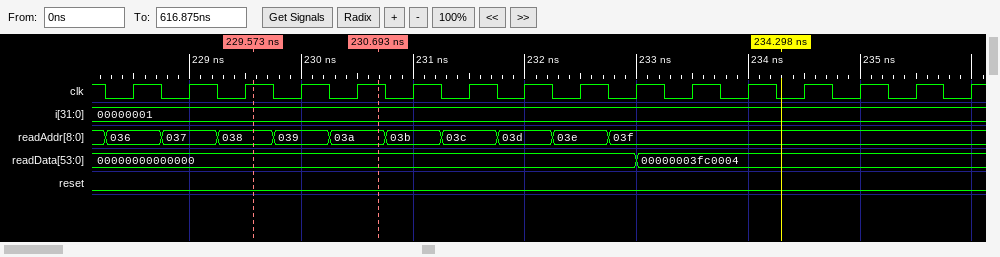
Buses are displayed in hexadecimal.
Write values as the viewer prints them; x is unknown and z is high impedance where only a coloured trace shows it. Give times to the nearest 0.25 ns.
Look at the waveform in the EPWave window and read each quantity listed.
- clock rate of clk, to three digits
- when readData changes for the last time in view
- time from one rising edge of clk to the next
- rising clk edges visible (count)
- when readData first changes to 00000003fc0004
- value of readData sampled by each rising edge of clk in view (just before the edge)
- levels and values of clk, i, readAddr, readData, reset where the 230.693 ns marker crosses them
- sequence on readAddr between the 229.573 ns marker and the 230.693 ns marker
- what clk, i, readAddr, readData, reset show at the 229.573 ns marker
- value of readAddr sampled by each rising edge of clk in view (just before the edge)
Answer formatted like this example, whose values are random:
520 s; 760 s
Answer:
2.00 GHz; 233 ns; 0.5 ns; 16; 233 ns; 00000000000000, 00000000000000, 00000000000000, 00000000000000, 00000000000000, 00000000000000, 00000000000000, 00000000000000, 00000000000000, 00000000000000, 00000003fc0004, 00000003fc0004, 00000003fc0004, 00000003fc0004, 00000003fc0004, 00000003fc0004; clk=1, i=00000001, readAddr=03a, readData=00000000000000, reset=0; 038, 039, 03a; clk=1, i=00000001, readAddr=038, readData=00000000000000, reset=0; 036, 037, 038, 039, 03a, 03b, 03c, 03d, 03e, 03f, 03f, 03f, 03f, 03f, 03f, 03f
